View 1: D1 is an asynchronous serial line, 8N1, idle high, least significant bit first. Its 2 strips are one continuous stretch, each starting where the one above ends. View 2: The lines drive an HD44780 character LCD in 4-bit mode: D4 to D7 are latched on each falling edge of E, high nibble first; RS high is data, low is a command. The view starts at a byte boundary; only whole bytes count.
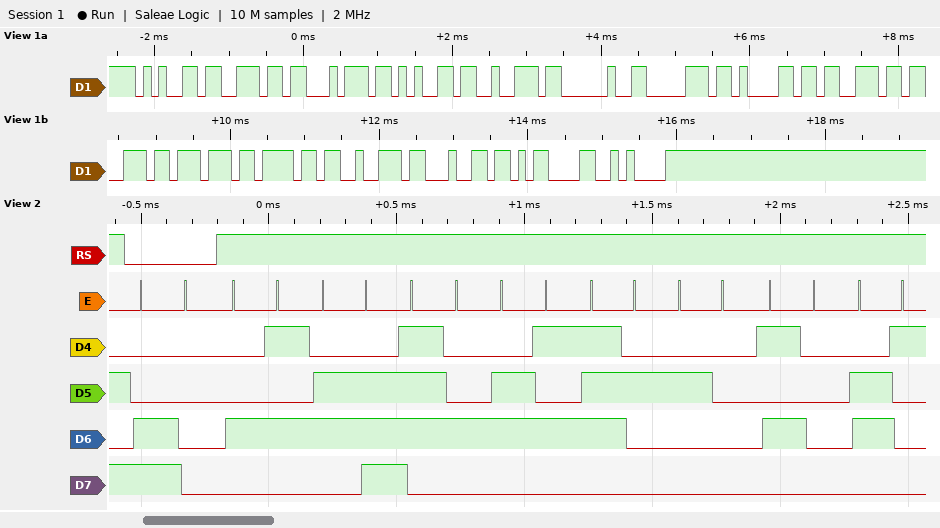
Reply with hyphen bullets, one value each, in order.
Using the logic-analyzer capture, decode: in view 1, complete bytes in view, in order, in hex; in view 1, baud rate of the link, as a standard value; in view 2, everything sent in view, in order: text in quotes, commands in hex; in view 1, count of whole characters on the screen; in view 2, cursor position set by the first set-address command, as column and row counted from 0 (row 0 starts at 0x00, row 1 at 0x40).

- 65 6E 74 65 72 20 70 61 73 73 77 6F 72 64 0D 0A
- 9600 baud
- 0xC0 "Enter Pa"
- 16
- column 0, row 1
